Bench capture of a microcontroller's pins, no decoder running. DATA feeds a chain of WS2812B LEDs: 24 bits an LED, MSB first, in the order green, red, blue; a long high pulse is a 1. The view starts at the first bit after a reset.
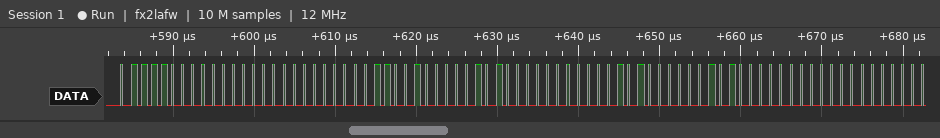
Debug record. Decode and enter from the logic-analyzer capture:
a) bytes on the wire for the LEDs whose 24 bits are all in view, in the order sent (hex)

78 00 00 64 14 00 50 28 00
